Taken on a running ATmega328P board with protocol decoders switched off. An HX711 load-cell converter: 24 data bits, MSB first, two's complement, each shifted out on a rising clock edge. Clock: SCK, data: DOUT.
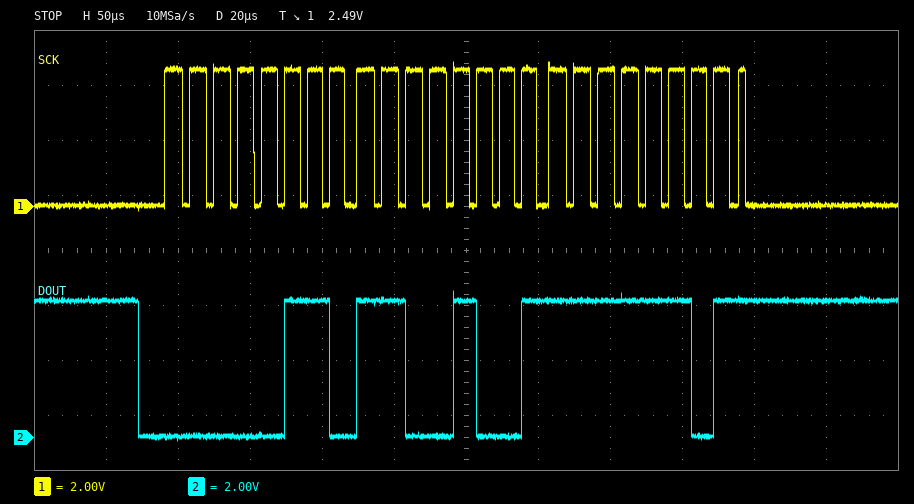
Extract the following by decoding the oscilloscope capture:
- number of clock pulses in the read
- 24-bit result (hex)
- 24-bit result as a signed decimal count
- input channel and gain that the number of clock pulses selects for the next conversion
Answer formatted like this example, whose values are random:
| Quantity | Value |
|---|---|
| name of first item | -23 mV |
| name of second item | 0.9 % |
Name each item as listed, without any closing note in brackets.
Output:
| Quantity | Value |
|---|---|
| number of clock pulses in the read | 25 |
| 24-bit result | 0x06C9FD |
| 24-bit result as a signed decimal count | 444925 |
| input channel and gain that the number of clock pulses selects for the next conversion | channel A, gain 128 |
